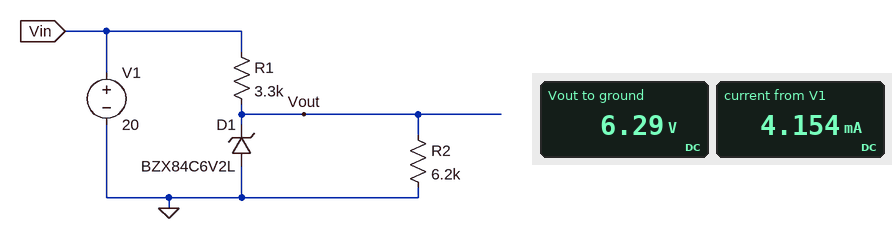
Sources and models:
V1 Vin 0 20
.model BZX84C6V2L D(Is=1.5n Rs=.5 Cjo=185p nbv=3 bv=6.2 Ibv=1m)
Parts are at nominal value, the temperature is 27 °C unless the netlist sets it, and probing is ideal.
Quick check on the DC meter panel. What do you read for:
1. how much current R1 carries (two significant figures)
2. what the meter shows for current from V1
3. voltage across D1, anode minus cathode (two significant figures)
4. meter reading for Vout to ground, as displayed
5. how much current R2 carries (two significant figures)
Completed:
4.2 mA
4.154 mA
-6.3 V
6.29 V
1.0 mA
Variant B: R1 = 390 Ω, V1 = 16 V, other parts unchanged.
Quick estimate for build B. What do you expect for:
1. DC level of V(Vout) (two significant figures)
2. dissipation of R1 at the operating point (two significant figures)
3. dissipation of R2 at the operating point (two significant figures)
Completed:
6.5 V
230 mW
6.7 mW
